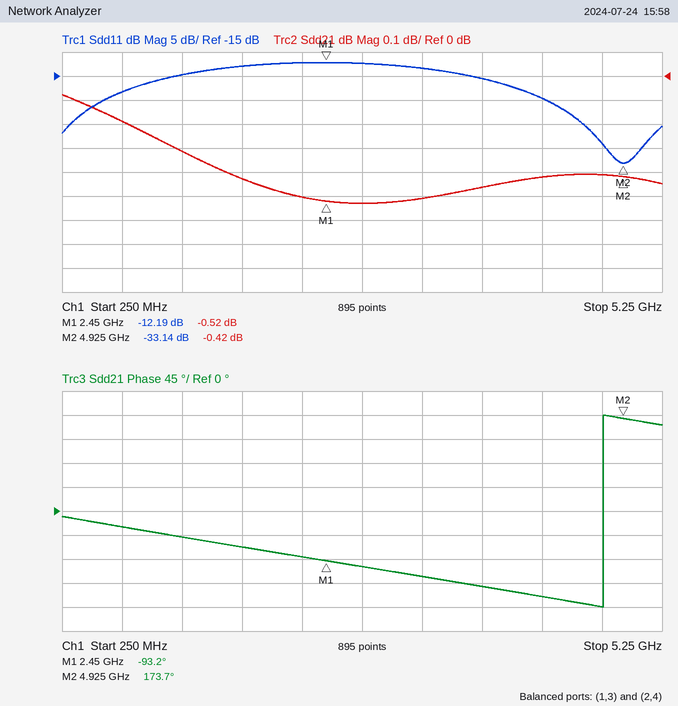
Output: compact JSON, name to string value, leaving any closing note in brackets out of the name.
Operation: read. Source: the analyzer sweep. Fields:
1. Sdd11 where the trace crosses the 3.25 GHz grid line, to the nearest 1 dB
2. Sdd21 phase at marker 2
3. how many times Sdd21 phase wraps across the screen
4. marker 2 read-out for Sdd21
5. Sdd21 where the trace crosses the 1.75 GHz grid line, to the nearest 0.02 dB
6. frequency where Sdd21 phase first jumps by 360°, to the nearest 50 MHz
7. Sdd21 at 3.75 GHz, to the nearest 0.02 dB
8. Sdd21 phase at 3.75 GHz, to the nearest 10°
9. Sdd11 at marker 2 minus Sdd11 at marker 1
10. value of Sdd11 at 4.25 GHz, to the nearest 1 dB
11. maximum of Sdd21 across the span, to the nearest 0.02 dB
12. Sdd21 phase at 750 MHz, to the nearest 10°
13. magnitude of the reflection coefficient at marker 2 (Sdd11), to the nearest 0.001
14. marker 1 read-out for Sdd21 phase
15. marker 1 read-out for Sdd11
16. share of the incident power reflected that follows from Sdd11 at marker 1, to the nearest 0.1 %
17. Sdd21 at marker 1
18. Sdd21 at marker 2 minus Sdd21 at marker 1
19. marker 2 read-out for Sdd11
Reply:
{"Sdd11 where the trace crosses the 3.25 GHz grid line, to the nearest 1 dB": "-13 dB", "Sdd21 phase at marker 2": "173.7°", "how many times Sdd21 phase wraps across the screen": "1", "marker 2 read-out for Sdd21": "-0.42 dB", "Sdd21 where the trace crosses the 1.75 GHz grid line, to the nearest 0.02 dB": "-0.42 dB", "frequency where Sdd21 phase first jumps by 360°, to the nearest 50 MHz": "4.75 GHz", "Sdd21 at 3.75 GHz, to the nearest 0.02 dB": "-0.46 dB", "Sdd21 phase at 3.75 GHz, to the nearest 10°": "-140°", "Sdd11 at marker 2 minus Sdd11 at marker 1": "-20.95 dB", "value of Sdd11 at 4.25 GHz, to the nearest 1 dB": "-20 dB", "maximum of Sdd21 across the span, to the nearest 0.02 dB": "-0.08 dB", "Sdd21 phase at 750 MHz, to the nearest 10°": "-30°", "magnitude of the reflection coefficient at marker 2 (Sdd11), to the nearest 0.001": "0.022", "marker 1 read-out for Sdd21 phase": "-93.2°", "marker 1 read-out for Sdd11": "-12.19 dB", "share of the incident power reflected that follows from Sdd11 at marker 1, to the nearest 0.1 %": "6.0 %", "Sdd21 at marker 1": "-0.52 dB", "Sdd21 at marker 2 minus Sdd21 at marker 1": "0.10 dB", "marker 2 read-out for Sdd11": "-33.14 dB"}
